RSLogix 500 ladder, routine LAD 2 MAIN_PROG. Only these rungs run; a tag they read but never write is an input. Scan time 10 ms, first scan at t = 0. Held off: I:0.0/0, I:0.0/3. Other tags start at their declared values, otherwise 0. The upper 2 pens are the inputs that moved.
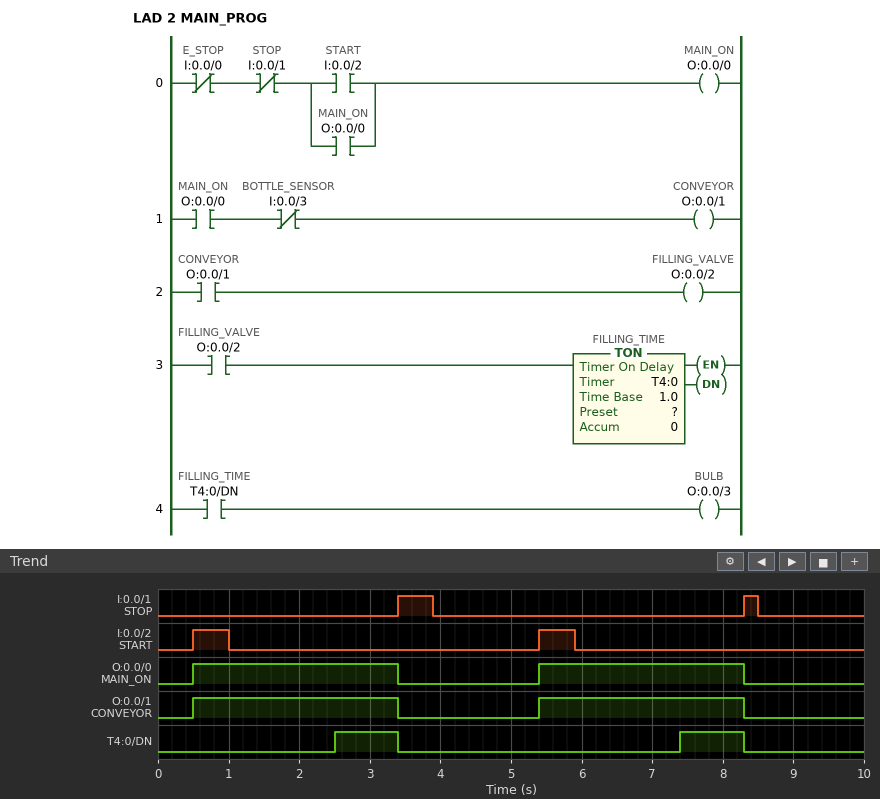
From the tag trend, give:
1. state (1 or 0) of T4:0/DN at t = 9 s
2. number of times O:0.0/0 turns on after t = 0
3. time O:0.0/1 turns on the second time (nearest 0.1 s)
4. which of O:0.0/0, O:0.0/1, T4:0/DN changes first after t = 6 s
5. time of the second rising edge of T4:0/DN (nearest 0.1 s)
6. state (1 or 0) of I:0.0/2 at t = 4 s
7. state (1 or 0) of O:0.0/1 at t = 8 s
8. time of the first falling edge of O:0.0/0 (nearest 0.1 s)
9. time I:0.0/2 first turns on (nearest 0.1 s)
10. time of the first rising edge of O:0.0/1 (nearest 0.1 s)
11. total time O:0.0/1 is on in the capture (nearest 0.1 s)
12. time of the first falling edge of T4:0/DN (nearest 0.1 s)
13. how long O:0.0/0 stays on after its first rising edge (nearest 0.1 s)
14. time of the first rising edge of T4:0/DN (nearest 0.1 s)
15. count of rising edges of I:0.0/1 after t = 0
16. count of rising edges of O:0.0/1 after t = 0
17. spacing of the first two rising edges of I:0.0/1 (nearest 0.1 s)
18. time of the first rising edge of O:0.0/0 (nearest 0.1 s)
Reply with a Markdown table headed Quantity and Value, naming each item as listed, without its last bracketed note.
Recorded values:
| Quantity | Value |
|---|---|
| state (1 or 0) of T4:0/DN at t = 9 s | 0 |
| number of times O:0.0/0 turns on after t = 0 | 2 |
| time O:0.0/1 turns on the second time | 5.4 s |
| which of O:0.0/0, O:0.0/1, T4:0/DN changes first after t = 6 s | T4:0/DN |
| time of the second rising edge of T4:0/DN | 7.4 s |
| state (1 or 0) of I:0.0/2 at t = 4 s | 0 |
| state (1 or 0) of O:0.0/1 at t = 8 s | 1 |
| time of the first falling edge of O:0.0/0 | 3.4 s |
| time I:0.0/2 first turns on | 0.5 s |
| time of the first rising edge of O:0.0/1 | 0.5 s |
| total time O:0.0/1 is on in the capture | 5.8 s |
| time of the first falling edge of T4:0/DN | 3.4 s |
| how long O:0.0/0 stays on after its first rising edge | 2.9 s |
| time of the first rising edge of T4:0/DN | 2.5 s |
| count of rising edges of I:0.0/1 after t = 0 | 2 |
| count of rising edges of O:0.0/1 after t = 0 | 2 |
| spacing of the first two rising edges of I:0.0/1 | 4.9 s |
| time of the first rising edge of O:0.0/0 | 0.5 s |
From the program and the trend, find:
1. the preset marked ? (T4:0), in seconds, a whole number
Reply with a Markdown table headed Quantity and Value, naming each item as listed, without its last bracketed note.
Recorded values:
| Quantity | Value |
|---|---|
| the preset marked ? (T4:0), in seconds, a whole number | 2 s |
